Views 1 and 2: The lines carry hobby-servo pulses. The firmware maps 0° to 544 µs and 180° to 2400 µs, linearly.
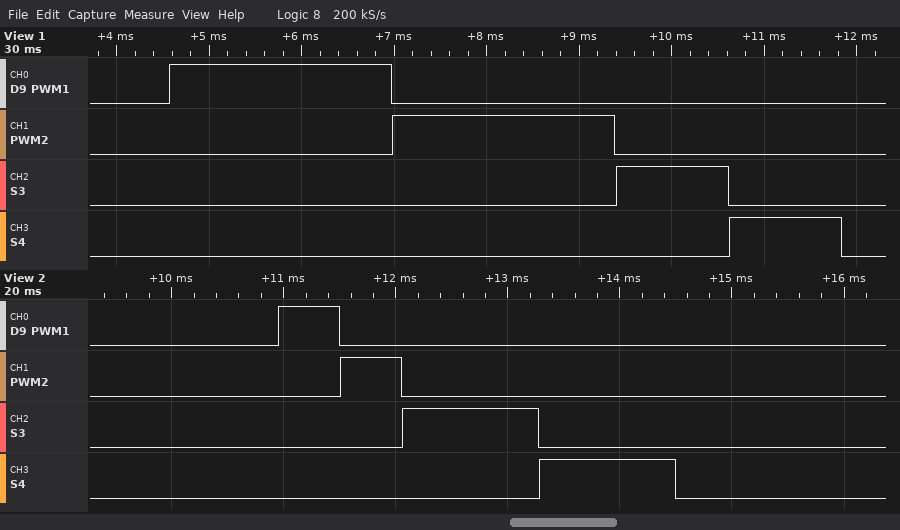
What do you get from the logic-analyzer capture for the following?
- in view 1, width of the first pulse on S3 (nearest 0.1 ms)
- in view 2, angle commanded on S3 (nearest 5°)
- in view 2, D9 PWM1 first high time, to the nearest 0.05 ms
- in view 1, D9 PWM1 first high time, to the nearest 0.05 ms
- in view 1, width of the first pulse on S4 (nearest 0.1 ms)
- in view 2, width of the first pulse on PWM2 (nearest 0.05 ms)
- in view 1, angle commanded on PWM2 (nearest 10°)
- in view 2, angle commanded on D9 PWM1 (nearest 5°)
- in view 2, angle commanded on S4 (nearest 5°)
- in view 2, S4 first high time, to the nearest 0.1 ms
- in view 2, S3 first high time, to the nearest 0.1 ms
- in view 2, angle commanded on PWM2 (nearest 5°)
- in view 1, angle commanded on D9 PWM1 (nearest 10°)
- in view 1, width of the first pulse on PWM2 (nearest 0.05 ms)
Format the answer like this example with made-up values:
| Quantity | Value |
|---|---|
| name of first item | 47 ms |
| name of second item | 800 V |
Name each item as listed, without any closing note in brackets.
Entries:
| Quantity | Value |
|---|---|
| in view 1, width of the first pulse on S3 | 1.2 ms |
| in view 2, angle commanded on S3 | 65° |
| in view 2, D9 PWM1 first high time, to the nearest 0.05 ms | 0.55 ms |
| in view 1, D9 PWM1 first high time, to the nearest 0.05 ms | 2.40 ms |
| in view 1, width of the first pulse on S4 | 1.2 ms |
| in view 2, width of the first pulse on PWM2 | 0.55 ms |
| in view 1, angle commanded on PWM2 | 180° |
| in view 2, angle commanded on D9 PWM1 | 0° |
| in view 2, angle commanded on S4 | 65° |
| in view 2, S4 first high time, to the nearest 0.1 ms | 1.2 ms |
| in view 2, S3 first high time, to the nearest 0.1 ms | 1.2 ms |
| in view 2, angle commanded on PWM2 | 0° |
| in view 1, angle commanded on D9 PWM1 | 180° |
| in view 1, width of the first pulse on PWM2 | 2.40 ms |
